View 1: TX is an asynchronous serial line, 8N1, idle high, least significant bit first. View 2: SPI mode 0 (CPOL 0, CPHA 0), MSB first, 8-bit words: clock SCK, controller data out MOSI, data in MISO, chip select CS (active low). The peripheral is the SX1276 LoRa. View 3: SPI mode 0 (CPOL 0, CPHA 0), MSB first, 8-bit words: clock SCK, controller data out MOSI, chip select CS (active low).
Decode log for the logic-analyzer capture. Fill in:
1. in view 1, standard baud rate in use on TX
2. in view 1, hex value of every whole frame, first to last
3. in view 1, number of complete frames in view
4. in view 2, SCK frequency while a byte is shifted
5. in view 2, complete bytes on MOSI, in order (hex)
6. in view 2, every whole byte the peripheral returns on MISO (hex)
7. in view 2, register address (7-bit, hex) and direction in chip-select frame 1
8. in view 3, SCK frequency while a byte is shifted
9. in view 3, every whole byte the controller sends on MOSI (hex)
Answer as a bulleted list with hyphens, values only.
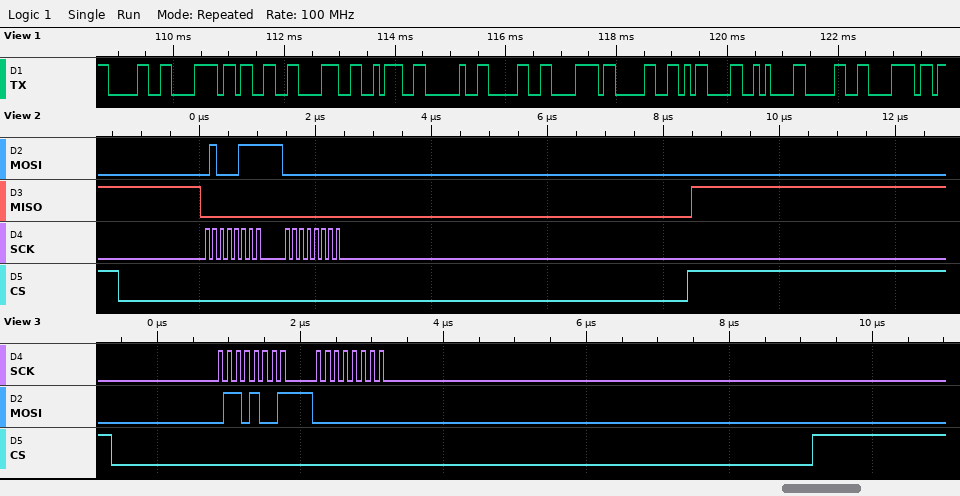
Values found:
- 9600 baud
- 30 78 33 38 3A 20 30 78 30 0D 0A 30 78
- 13
- 8 MHz
- 47 00
- 00 00
- 0x47 read
- 8 MHz
- 69 00
